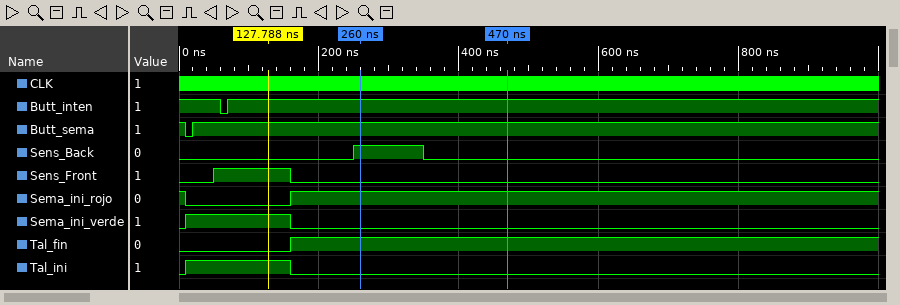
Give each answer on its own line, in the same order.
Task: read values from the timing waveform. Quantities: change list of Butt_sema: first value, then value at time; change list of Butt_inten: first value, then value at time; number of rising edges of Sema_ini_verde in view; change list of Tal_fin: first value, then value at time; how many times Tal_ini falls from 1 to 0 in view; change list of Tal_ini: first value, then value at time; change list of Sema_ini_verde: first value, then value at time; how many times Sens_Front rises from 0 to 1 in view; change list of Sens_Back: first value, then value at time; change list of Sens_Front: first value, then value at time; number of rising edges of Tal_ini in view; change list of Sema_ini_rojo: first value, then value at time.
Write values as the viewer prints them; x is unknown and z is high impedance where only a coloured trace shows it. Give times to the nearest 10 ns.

1, 0 at 10 ns, 1 at 20 ns
1, 0 at 60 ns, 1 at 70 ns
1
0, 1 at 160 ns
1
0, 1 at 10 ns, 0 at 160 ns
0, 1 at 10 ns, 0 at 160 ns
1
0, 1 at 250 ns, 0 at 350 ns
0, 1 at 50 ns, 0 at 160 ns
1
1, 0 at 10 ns, 1 at 160 ns
